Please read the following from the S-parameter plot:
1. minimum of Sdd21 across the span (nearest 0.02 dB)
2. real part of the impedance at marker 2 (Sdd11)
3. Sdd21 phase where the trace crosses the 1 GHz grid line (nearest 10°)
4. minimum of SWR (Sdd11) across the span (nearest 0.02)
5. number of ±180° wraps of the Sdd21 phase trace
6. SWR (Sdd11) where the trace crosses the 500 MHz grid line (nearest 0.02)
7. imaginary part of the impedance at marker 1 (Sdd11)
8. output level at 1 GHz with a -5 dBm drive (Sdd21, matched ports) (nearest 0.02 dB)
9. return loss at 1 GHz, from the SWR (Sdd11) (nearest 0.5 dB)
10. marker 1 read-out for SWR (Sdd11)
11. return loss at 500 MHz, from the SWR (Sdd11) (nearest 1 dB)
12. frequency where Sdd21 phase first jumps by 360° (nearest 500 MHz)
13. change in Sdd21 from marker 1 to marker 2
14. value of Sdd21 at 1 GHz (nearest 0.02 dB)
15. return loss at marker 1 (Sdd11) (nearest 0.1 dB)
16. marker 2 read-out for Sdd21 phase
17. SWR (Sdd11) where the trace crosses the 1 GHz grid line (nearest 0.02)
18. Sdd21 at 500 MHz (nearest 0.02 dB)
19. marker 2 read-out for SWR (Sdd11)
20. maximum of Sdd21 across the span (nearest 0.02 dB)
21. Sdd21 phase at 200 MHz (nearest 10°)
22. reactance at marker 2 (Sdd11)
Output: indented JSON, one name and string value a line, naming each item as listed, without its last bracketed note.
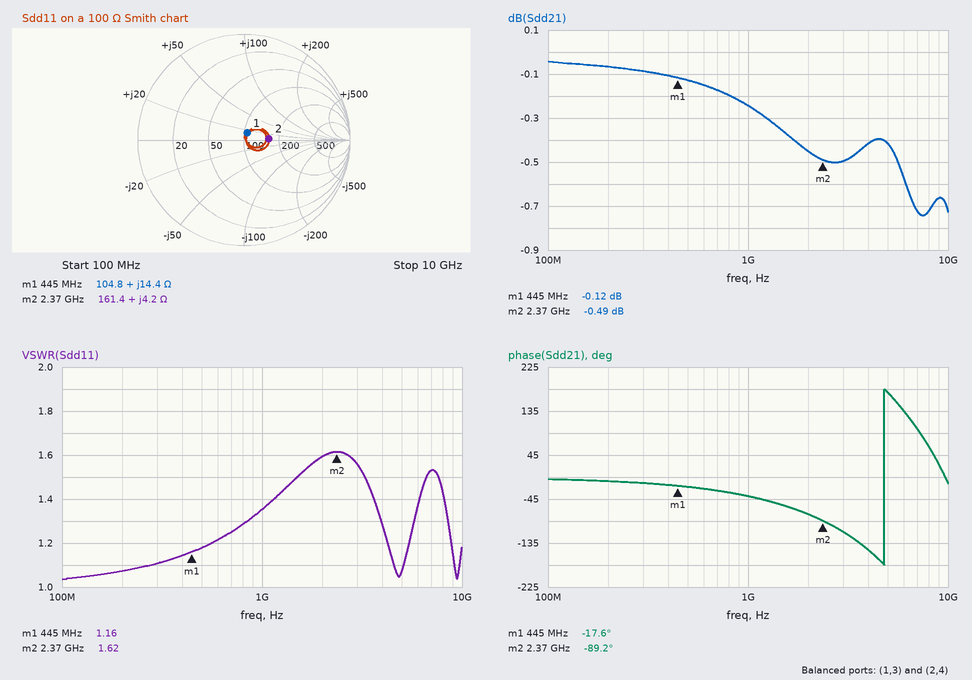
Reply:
{
  "minimum of Sdd21 across the span": "-0.74 dB",
  "real part of the impedance at marker 2": "161.4 Ω",
  "Sdd21 phase where the trace crosses the 1 GHz grid line": "-40°",
  "minimum of SWR (Sdd11) across the span": "1.04",
  "number of ±180° wraps of the Sdd21 phase trace": "1",
  "SWR (Sdd11) where the trace crosses the 500 MHz grid line": "1.18",
  "imaginary part of the impedance at marker 1": "+14.4 Ω",
  "output level at 1 GHz with a -5 dBm drive (Sdd21, matched ports)": "-5.24 dBm",
  "return loss at 1 GHz, from the SWR (Sdd11)": "16.5 dB",
  "marker 1 read-out for SWR": "1.16",
  "return loss at 500 MHz, from the SWR (Sdd11)": "22 dB",
  "frequency where Sdd21 phase first jumps by 360°": "5.0 GHz",
  "change in Sdd21 from marker 1 to marker 2": "-0.37 dB",
  "value of Sdd21 at 1 GHz": "-0.24 dB",
  "return loss at marker 1 (Sdd11)": "22.6 dB",
  "marker 2 read-out for Sdd21 phase": "-89.2°",
  "SWR (Sdd11) where the trace crosses the 1 GHz grid line": "1.36",
  "Sdd21 at 500 MHz": "-0.12 dB",
  "marker 2 read-out for SWR": "1.62",
  "maximum of Sdd21 across the span": "-0.04 dB",
  "Sdd21 phase at 200 MHz": "-10°",
  "reactance at marker 2": "+4.2 Ω"
}
